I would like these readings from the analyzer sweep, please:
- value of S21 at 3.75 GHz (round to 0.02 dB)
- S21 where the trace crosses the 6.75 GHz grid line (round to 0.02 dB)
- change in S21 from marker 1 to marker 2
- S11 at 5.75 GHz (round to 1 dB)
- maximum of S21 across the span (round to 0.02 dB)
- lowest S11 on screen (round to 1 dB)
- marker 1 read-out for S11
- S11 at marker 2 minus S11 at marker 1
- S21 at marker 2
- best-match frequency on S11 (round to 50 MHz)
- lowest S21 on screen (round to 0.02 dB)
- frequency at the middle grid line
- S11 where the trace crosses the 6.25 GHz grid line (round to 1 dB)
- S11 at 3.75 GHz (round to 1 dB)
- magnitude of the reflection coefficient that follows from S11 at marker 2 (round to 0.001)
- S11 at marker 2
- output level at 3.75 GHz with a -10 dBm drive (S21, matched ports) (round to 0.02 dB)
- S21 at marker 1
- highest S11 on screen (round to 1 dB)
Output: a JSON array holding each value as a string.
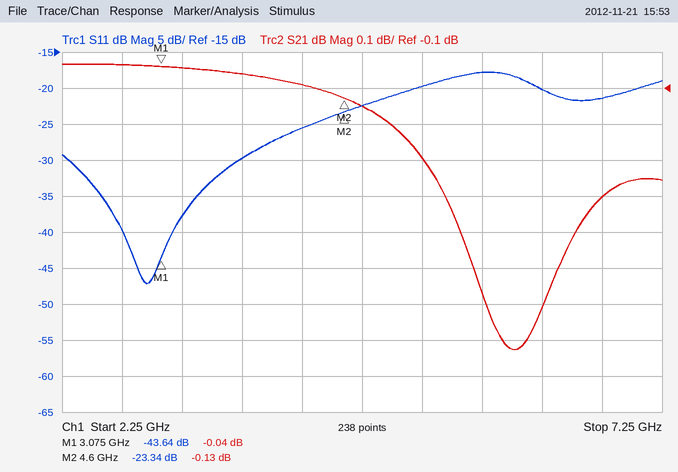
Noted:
["-0.06 dB", "-0.40 dB", "-0.09 dB", "-18 dB", "-0.04 dB", "-47 dB", "-43.64 dB", "20.30 dB", "-0.13 dB", "2.95 GHz", "-0.82 dB", "4.75 GHz", "-20 dB", "-30 dB", "0.068", "-23.34 dB", "-10.06 dBm", "-0.04 dB", "-18 dB"]
